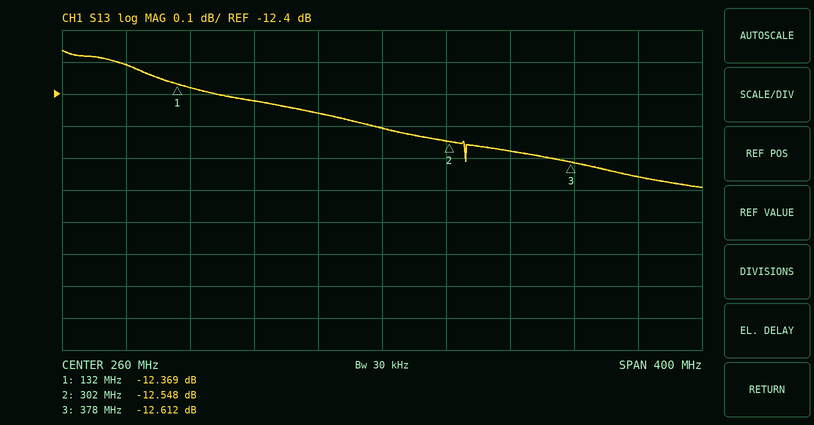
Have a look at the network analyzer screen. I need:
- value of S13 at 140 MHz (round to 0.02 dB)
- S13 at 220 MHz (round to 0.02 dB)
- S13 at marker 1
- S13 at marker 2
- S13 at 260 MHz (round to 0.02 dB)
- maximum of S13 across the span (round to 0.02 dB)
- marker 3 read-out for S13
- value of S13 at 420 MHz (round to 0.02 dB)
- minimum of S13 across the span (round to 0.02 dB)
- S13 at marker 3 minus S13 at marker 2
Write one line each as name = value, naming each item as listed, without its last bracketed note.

value of S13 at 140 MHz = -12.38 dB
S13 at 220 MHz = -12.46 dB
S13 at marker 1 = -12.369 dB
S13 at marker 2 = -12.548 dB
S13 at 260 MHz = -12.50 dB
maximum of S13 across the span = -12.26 dB
marker 3 read-out for S13 = -12.612 dB
value of S13 at 420 MHz = -12.66 dB
minimum of S13 across the span = -12.70 dB
S13 at marker 3 minus S13 at marker 2 = -0.064 dB
